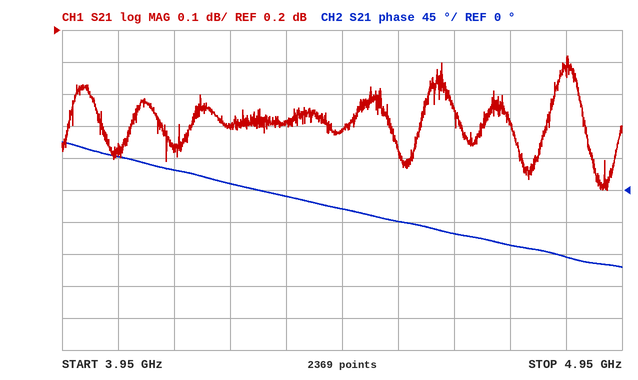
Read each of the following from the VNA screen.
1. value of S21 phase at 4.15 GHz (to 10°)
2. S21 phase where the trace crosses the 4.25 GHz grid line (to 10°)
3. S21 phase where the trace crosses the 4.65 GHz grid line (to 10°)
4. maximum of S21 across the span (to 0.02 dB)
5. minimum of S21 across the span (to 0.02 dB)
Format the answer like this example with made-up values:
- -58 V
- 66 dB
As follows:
- 30°
- 10°
- -60°
- 0.12 dB
- -0.30 dB
